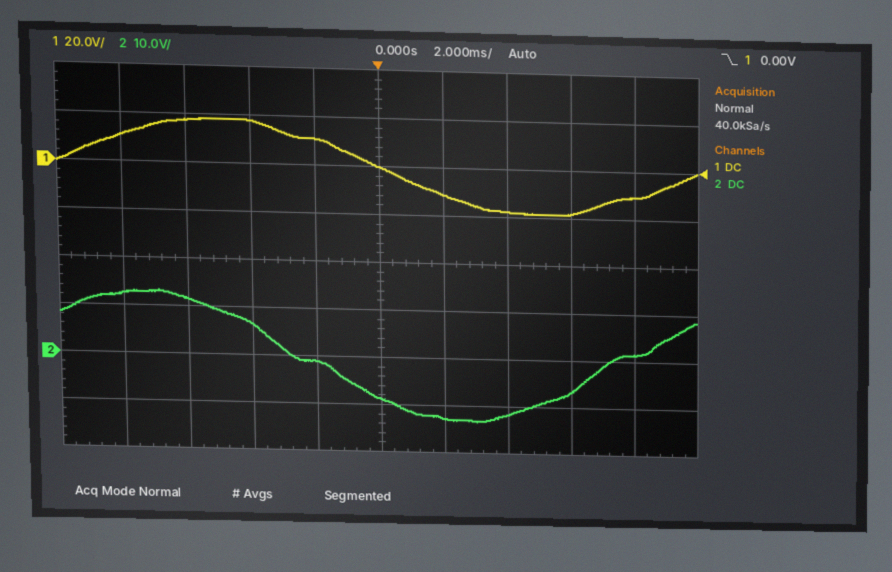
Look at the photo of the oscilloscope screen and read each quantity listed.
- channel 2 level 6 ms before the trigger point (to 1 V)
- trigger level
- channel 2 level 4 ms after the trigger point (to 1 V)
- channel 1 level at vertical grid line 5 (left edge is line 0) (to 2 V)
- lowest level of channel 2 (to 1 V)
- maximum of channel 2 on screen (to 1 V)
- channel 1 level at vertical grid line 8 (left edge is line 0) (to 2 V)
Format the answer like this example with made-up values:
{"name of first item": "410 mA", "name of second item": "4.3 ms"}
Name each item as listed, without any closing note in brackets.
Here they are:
{"channel 2 level 6 ms before the trigger point": "12 V", "trigger level": "0.00 V", "channel 2 level 4 ms after the trigger point": "-12 V", "channel 1 level at vertical grid line 5 (left edge is line 0)": "0 V", "lowest level of channel 2": "-13 V", "maximum of channel 2 on screen": "13 V", "channel 1 level at vertical grid line 8 (left edge is line 0)": "-18 V"}
